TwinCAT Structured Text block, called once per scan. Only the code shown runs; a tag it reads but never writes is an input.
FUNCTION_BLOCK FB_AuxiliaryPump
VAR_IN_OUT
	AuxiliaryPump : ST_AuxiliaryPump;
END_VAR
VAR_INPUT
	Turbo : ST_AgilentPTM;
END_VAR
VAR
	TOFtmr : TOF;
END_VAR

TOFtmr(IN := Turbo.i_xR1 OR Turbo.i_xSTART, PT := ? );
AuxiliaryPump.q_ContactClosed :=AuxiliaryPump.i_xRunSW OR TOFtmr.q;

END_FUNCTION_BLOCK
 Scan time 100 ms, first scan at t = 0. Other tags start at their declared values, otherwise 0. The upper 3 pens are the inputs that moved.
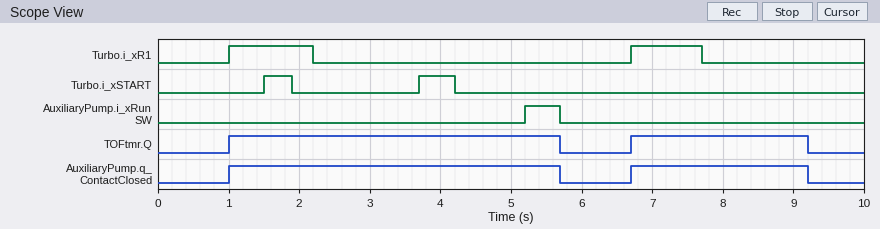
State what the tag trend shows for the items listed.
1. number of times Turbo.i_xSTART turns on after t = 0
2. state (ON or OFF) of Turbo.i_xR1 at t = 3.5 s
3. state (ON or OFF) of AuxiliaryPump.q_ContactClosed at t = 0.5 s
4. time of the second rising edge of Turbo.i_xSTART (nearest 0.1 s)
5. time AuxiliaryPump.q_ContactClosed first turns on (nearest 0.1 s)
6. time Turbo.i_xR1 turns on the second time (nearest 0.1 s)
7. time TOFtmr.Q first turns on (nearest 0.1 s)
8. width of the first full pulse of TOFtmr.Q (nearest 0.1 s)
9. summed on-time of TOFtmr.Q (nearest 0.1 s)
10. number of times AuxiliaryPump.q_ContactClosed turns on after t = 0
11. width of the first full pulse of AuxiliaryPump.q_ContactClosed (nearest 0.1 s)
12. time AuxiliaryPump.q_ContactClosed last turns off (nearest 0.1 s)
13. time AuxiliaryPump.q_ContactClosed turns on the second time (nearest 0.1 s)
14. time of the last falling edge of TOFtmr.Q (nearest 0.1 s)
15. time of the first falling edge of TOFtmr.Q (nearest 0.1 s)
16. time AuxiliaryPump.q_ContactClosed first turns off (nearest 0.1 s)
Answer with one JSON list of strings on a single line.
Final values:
["2", "OFF", "OFF", "3.7 s", "1.0 s", "6.7 s", "1.0 s", "4.7 s", "7.2 s", "2", "4.7 s", "9.2 s", "6.7 s", "9.2 s", "5.7 s", "5.7 s"]
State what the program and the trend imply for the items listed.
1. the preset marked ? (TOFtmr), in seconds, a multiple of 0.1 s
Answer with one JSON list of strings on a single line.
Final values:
["1.5 s"]
